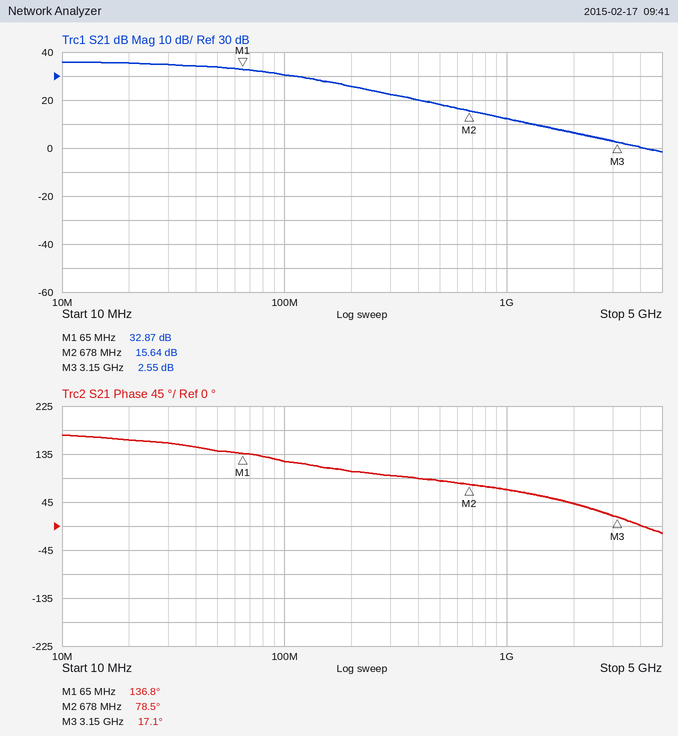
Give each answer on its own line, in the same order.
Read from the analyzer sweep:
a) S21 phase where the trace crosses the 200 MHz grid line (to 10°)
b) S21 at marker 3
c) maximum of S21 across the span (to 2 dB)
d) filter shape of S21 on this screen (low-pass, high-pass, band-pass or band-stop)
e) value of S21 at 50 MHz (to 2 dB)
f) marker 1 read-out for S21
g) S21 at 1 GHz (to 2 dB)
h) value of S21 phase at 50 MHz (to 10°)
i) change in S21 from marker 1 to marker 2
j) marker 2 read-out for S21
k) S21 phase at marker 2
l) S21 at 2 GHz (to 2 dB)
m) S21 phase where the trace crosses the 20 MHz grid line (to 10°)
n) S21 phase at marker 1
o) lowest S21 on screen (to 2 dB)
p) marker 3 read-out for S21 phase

100°
2.55 dB
36 dB
low-pass
34 dB
32.87 dB
12 dB
140°
-17.23 dB
15.64 dB
78.5°
6 dB
160°
136.8°
-2 dB
17.1°
